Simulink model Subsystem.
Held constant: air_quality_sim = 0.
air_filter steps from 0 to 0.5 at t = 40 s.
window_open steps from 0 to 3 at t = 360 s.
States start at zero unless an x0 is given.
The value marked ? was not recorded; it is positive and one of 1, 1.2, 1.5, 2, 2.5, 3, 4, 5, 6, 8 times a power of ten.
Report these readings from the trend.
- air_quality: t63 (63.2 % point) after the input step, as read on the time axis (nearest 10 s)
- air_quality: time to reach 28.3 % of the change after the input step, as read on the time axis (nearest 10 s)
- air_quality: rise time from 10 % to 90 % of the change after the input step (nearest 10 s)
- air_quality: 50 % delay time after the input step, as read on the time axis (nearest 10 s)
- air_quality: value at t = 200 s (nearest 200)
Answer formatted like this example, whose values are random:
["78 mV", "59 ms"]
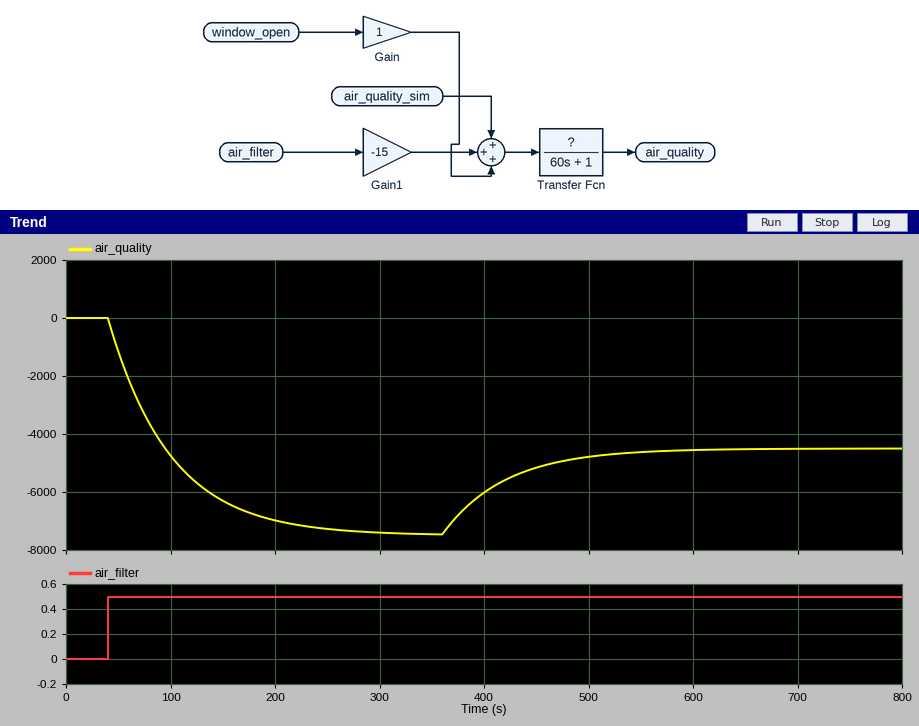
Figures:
["100 s", "60 s", "130 s", "80 s", "-7000"]
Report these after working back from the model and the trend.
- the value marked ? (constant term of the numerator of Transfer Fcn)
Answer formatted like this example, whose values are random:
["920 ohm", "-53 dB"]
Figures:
["1000"]
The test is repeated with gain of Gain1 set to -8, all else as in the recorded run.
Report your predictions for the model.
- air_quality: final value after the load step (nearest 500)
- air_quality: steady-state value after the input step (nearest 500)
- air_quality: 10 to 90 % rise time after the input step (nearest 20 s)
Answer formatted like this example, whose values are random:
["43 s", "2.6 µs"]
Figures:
["-1000", "-4000", "140 s"]
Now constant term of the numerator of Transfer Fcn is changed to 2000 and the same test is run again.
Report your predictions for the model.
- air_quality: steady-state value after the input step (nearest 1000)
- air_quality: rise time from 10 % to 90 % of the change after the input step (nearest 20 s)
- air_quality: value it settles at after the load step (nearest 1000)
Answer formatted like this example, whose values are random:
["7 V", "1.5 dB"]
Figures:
["-15000", "140 s", "-9000"]
